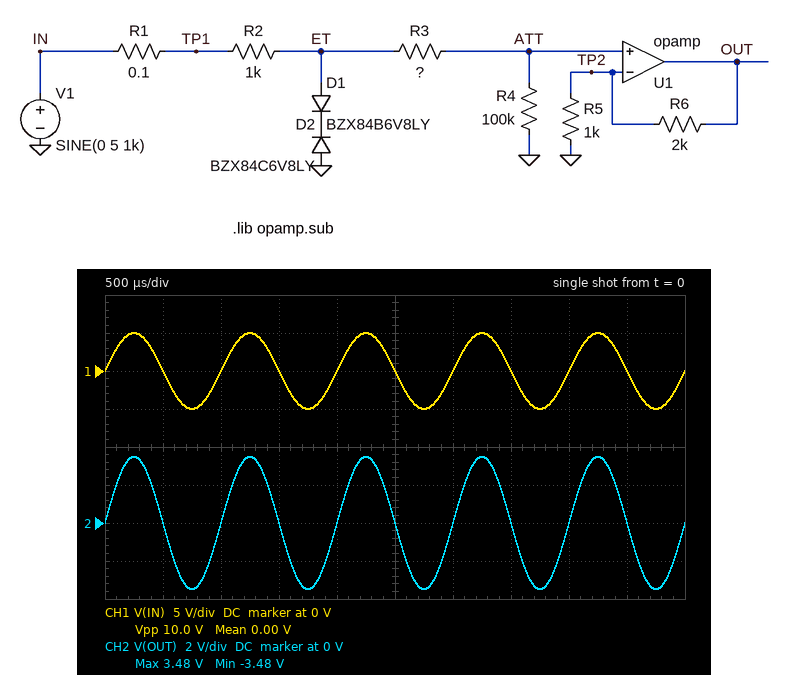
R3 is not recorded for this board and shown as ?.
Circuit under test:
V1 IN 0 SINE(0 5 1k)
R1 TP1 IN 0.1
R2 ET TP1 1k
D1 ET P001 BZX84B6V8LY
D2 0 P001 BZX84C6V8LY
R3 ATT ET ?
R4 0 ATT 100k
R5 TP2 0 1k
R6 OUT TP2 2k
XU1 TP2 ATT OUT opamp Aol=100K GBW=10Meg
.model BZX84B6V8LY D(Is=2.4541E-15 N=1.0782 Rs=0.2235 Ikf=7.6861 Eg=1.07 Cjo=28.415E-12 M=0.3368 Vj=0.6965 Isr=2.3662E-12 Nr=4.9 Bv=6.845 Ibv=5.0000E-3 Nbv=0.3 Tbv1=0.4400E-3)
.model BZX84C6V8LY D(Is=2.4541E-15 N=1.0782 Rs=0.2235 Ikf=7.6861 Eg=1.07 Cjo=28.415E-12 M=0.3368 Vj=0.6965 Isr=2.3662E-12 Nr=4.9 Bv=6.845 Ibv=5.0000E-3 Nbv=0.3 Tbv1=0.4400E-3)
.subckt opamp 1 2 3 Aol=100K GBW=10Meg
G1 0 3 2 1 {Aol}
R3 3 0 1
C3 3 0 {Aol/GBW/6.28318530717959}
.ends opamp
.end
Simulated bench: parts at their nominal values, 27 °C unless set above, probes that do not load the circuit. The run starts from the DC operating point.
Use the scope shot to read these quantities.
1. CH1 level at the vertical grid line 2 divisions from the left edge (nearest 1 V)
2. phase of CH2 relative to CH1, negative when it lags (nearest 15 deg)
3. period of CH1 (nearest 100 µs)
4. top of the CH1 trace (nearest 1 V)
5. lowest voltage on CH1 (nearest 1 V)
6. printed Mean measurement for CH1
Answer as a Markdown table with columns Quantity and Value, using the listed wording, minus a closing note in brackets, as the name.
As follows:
| Quantity | Value |
|---|---|
| CH1 level at the vertical grid line 2 divisions from the left edge | 0 V |
| phase of CH2 relative to CH1, negative when it lags | 0 deg |
| period of CH1 | 1.0 ms |
| top of the CH1 trace | 5 V |
| lowest voltage on CH1 | -5 V |
| printed Mean measurement for CH1 | 0.00 V |
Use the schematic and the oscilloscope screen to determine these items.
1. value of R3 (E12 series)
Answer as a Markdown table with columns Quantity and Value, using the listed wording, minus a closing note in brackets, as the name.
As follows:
| Quantity | Value |
|---|---|
| value of R3 | 330 kΩ |
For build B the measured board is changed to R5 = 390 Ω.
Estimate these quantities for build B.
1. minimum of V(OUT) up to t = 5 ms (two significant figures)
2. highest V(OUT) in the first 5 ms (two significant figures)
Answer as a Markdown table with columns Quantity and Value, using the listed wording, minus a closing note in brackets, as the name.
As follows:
| Quantity | Value |
|---|---|
| minimum of V(OUT) up to t = 5 ms | -7.1 V |
| highest V(OUT) in the first 5 ms | 7.1 V |
